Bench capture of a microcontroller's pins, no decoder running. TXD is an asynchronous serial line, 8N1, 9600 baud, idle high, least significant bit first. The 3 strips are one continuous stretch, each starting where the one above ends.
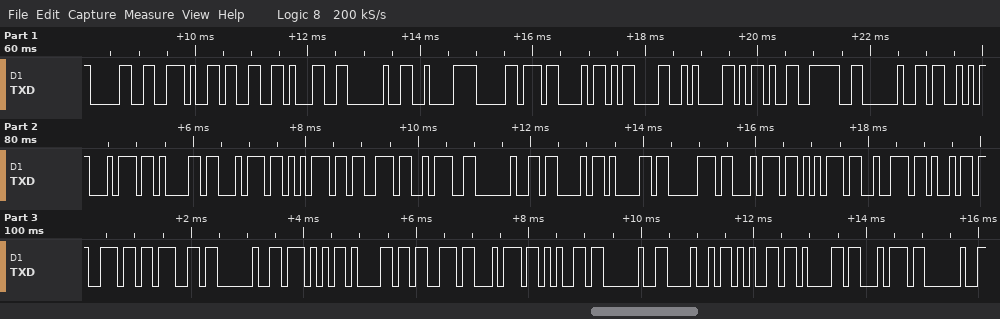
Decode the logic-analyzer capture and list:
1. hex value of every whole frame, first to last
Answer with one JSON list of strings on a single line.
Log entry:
["0x30 0x2E 0x33 0x31 0x20 0xC2 0xB0 0x43 0x0D 0x0A 0x2D 0x3E 0x20 0x53 0x74 0x61 0x74 0x75 0x73 0x3A 0x20 0x43 0x61 0x70 0x74 0x75 0x72 0x69 0x6E 0x67 0x20 0x57 0x61 0x73 0x74 0x65 0x20 0x48 0x65 0x61 0x74 0x20"]
